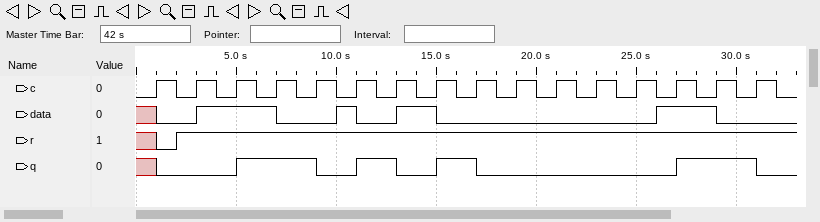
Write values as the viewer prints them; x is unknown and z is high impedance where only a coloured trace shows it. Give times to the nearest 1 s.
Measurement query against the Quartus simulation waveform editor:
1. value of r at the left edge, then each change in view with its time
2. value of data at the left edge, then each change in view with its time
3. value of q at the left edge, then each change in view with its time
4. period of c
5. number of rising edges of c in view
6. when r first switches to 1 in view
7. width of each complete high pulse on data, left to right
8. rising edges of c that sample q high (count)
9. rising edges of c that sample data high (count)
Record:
x, 0 at 1 s, 1 at 2 s
x, 0 at 1 s, 1 at 3 s, 0 at 7 s, 1 at 10 s, 0 at 11 s, 1 at 13 s, 0 at 15 s, 1 at 26 s, 0 at 29 s
x, 0 at 1 s, 1 at 5 s, 0 at 9 s, 1 at 11 s, 0 at 13 s, 1 at 15 s, 0 at 17 s, 1 at 27 s, 0 at 31 s
2 s
16
2 s
4 s, 1 s, 2 s, 3 s
6
6
